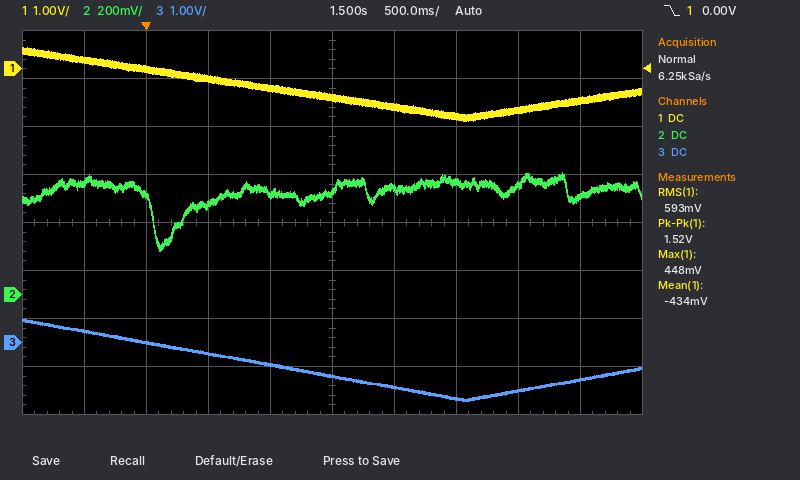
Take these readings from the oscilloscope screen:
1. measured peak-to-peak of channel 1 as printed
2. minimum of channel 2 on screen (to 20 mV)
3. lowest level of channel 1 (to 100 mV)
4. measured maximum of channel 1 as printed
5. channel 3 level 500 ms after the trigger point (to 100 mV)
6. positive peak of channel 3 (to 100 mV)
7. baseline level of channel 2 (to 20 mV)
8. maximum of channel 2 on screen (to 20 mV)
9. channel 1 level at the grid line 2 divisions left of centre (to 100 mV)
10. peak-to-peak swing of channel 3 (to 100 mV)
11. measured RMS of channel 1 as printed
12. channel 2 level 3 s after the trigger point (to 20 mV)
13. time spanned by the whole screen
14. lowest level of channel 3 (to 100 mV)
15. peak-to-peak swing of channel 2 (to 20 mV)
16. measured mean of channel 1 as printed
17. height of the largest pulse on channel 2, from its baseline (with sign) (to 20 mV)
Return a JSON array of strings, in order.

["1.52 V", "180 mV", "-1.1 V", "448 mV", "-200 mV", "500 mV", "440 mV", "500 mV", "-200 mV", "1.7 V", "593 mV", "460 mV", "5 s", "-1.2 V", "320 mV", "-434 mV", "-260 mV"]
